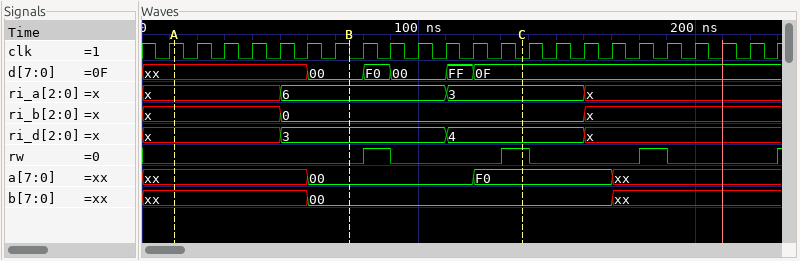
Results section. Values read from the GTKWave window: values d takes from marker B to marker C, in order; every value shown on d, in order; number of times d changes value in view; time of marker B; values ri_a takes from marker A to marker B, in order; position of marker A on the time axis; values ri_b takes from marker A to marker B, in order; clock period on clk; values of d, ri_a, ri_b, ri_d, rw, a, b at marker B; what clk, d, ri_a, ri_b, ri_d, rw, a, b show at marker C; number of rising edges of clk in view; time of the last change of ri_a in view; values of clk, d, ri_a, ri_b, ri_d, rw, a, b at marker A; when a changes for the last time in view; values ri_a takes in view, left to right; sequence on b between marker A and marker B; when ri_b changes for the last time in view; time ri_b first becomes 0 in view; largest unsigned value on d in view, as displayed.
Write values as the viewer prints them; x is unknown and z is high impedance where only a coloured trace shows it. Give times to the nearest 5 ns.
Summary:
00, F0, 00, FF, 0F
xx, 00, F0, 00, FF, 0F
5
75 ns
x, 6
10 ns
x, 0
10 ns
d=00, ri_a=6, ri_b=0, ri_d=3, rw=0, a=00, b=00
clk=0, d=0F, ri_a=3, ri_b=0, ri_d=4, rw=1, a=F0, b=00
23
160 ns
clk=1, d=xx, ri_a=x, ri_b=x, ri_d=x, rw=0, a=xx, b=xx
170 ns
x, 6, 3, x
xx, 00
160 ns
50 ns
FF
